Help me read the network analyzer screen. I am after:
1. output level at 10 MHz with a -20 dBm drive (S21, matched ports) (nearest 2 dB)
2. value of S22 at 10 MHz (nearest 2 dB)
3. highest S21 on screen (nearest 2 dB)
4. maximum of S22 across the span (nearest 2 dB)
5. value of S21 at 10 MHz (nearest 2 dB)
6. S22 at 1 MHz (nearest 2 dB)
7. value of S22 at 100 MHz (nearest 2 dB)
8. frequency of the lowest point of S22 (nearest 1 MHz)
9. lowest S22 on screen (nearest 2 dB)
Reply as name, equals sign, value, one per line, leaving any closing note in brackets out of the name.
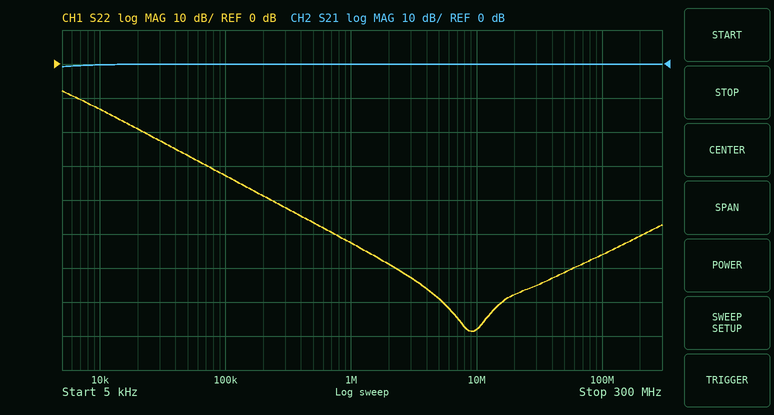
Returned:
output level at 10 MHz with a -20 dBm drive (S21, matched ports) = -20 dBm
value of S22 at 10 MHz = -78 dB
highest S21 on screen = 0 dB
maximum of S22 across the span = -8 dB
value of S21 at 10 MHz = 0 dB
S22 at 1 MHz = -52 dB
value of S22 at 100 MHz = -56 dB
frequency of the lowest point of S22 = 9 MHz
lowest S22 on screen = -78 dB
